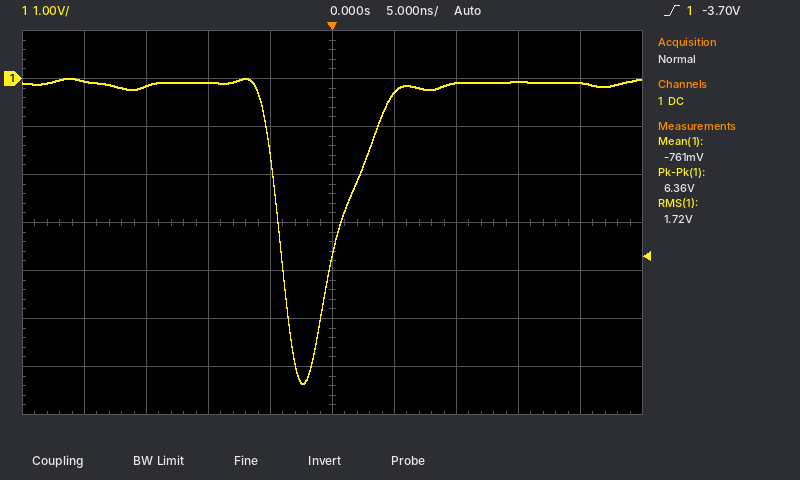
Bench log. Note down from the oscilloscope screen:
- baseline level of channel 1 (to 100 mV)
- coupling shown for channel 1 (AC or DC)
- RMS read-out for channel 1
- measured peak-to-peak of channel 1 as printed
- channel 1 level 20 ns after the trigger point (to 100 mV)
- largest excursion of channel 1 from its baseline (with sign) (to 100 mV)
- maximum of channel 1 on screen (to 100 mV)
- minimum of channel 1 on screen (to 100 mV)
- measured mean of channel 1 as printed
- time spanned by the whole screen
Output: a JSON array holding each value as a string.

["-100 mV", "DC", "1.72 V", "6.36 V", "-100 mV", "-6.3 V", "0.0 V", "-6.4 V", "-761 mV", "50 ns"]
